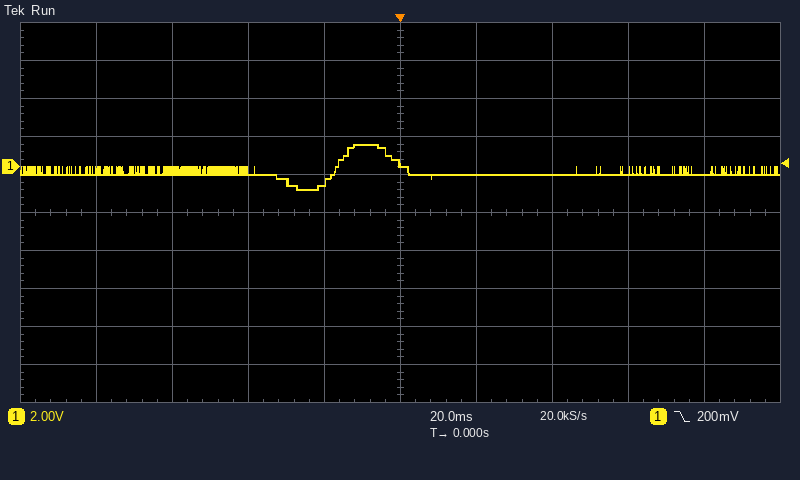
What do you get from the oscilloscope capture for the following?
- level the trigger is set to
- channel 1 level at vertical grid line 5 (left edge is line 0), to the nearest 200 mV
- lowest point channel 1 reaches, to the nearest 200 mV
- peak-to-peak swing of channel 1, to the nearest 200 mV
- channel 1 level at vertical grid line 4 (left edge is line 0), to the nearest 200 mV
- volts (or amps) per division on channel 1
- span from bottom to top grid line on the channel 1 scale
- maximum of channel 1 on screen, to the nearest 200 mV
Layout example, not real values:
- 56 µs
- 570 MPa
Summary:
- 200 mV
- 200 mV
- -1.2 V
- 2.4 V
- -800 mV
- 2 V
- 20 V
- 1.2 V
